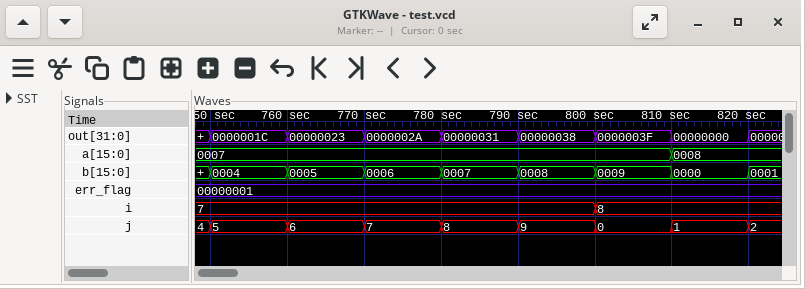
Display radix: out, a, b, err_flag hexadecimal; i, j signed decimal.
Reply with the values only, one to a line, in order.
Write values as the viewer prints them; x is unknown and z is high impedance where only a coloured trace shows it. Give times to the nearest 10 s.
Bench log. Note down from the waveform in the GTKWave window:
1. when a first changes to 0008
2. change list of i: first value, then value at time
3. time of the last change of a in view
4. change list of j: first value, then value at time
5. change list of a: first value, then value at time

810 s
7, 8 at 800 s
810 s
4, 5 at 750 s, 6 at 760 s, 7 at 770 s, 8 at 780 s, 9 at 790 s, 0 at 800 s, 1 at 810 s, 2 at 820 s
0007, 0008 at 810 s
